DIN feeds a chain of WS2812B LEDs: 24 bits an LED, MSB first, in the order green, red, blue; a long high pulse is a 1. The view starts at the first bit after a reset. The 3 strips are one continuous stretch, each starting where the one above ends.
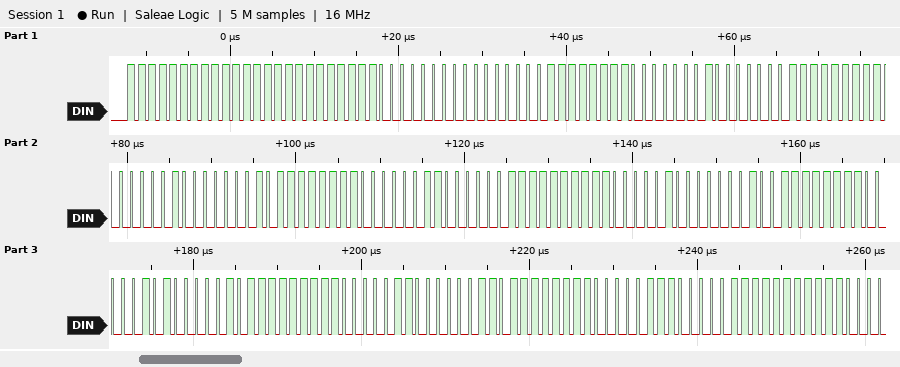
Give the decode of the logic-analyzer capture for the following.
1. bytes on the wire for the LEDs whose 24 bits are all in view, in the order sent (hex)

FF FF FF 00 00 FF 01 01 FF 02 02 FF 03 03 FF 04 04 FF 05 05 FF 06 06 FF 07 07 FF
